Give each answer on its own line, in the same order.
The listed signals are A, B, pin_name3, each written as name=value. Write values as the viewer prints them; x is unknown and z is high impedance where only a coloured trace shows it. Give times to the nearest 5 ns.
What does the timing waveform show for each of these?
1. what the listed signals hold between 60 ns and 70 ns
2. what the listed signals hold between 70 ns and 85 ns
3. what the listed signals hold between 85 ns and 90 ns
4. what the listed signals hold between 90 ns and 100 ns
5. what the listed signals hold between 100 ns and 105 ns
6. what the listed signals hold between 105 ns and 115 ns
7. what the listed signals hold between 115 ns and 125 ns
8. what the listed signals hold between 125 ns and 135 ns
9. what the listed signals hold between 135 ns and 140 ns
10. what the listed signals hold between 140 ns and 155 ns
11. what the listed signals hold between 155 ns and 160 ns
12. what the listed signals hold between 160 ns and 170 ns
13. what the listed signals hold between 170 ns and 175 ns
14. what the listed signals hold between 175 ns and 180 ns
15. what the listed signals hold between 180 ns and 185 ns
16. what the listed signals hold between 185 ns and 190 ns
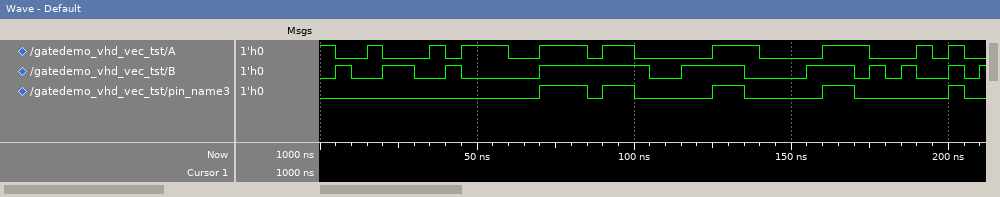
A=0, B=0, pin_name3=0
A=1, B=1, pin_name3=1
A=0, B=1, pin_name3=0
A=1, B=1, pin_name3=1
A=0, B=1, pin_name3=0
A=0, B=0, pin_name3=0
A=0, B=1, pin_name3=0
A=1, B=1, pin_name3=1
A=1, B=0, pin_name3=0
A=0, B=0, pin_name3=0
A=0, B=1, pin_name3=0
A=1, B=1, pin_name3=1
A=1, B=0, pin_name3=0
A=0, B=1, pin_name3=0
A=0, B=0, pin_name3=0
A=0, B=1, pin_name3=0
